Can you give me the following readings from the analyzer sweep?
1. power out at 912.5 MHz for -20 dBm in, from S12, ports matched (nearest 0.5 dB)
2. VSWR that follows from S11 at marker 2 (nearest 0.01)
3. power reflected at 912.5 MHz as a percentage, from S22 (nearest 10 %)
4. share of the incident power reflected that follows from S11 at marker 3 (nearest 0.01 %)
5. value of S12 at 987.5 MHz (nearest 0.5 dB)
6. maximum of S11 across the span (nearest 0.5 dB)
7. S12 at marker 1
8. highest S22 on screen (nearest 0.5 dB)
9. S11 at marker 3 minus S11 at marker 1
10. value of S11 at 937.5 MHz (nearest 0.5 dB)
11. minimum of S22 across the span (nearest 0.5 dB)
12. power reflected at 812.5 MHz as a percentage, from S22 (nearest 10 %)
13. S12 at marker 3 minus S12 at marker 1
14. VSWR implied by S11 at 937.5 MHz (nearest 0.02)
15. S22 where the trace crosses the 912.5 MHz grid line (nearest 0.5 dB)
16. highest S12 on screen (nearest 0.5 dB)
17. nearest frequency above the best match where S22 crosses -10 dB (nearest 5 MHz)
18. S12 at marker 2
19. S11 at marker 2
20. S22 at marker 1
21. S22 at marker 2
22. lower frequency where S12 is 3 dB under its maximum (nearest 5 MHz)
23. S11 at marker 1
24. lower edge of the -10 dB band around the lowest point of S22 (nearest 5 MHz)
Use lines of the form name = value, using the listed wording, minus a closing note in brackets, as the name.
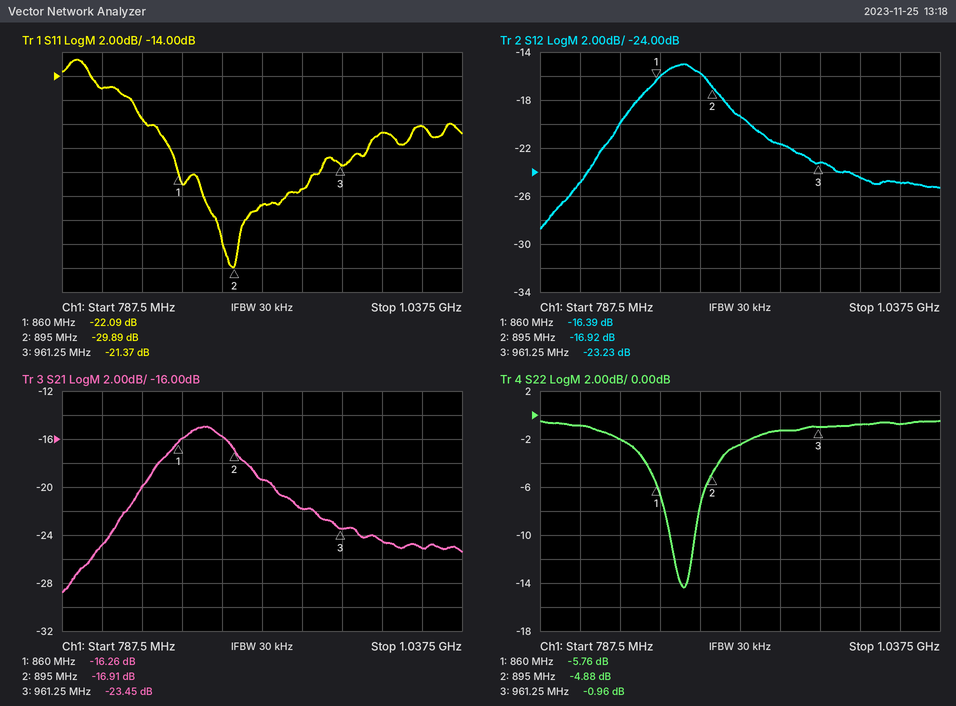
power out at 912.5 MHz for -20 dBm in, from S12, ports matched = -39.5 dBm
VSWR that follows from S11 at marker 2 = 1.07
power reflected at 912.5 MHz as a percentage, from S22 = 60 %
share of the incident power reflected that follows from S11 at marker 3 = 0.73 %
value of S12 at 987.5 MHz = -24.5 dB
maximum of S11 across the span = -12.5 dB
S12 at marker 1 = -16.39 dB
highest S22 on screen = -0.5 dB
S11 at marker 3 minus S11 at marker 1 = 0.72 dB
value of S11 at 937.5 MHz = -23.5 dB
minimum of S22 across the span = -14.5 dB
power reflected at 812.5 MHz as a percentage, from S22 = 80 %
S12 at marker 3 minus S12 at marker 1 = -6.84 dB
VSWR implied by S11 at 937.5 MHz = 1.14
S22 where the trace crosses the 912.5 MHz grid line = -2.5 dB
highest S12 on screen = -15.0 dB
nearest frequency above the best match where S22 crosses -10 dB = 885 MHz
S12 at marker 2 = -16.92 dB
S11 at marker 2 = -29.89 dB
S22 at marker 1 = -5.76 dB
S22 at marker 2 = -4.88 dB
lower frequency where S12 is 3 dB under its maximum = 850 MHz
S11 at marker 1 = -22.09 dB
lower edge of the -10 dB band around the lowest point of S22 = 870 MHz
